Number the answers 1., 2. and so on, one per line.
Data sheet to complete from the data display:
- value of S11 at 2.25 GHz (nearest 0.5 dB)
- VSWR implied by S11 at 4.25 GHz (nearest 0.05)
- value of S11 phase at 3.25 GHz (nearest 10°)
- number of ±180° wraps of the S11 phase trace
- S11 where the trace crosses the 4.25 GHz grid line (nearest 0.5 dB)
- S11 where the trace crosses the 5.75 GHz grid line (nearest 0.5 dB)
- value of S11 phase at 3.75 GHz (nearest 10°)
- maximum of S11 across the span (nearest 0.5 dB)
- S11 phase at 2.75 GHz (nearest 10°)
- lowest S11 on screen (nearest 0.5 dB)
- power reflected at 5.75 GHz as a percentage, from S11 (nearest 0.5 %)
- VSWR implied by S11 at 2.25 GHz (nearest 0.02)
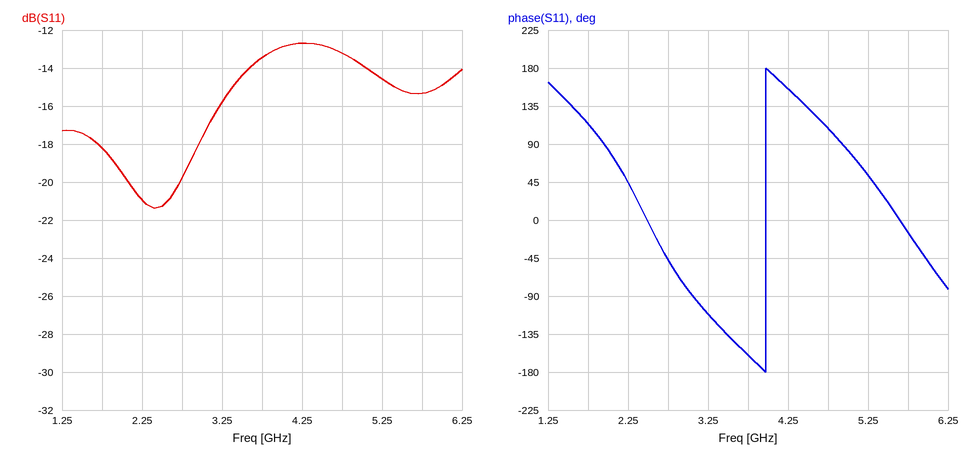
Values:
1. -21.0 dB
2. 1.60
3. -110°
4. 1
5. -12.5 dB
6. -15.5 dB
7. -160°
8. -12.5 dB
9. -50°
10. -21.5 dB
11. 3.0 %
12. 1.20
